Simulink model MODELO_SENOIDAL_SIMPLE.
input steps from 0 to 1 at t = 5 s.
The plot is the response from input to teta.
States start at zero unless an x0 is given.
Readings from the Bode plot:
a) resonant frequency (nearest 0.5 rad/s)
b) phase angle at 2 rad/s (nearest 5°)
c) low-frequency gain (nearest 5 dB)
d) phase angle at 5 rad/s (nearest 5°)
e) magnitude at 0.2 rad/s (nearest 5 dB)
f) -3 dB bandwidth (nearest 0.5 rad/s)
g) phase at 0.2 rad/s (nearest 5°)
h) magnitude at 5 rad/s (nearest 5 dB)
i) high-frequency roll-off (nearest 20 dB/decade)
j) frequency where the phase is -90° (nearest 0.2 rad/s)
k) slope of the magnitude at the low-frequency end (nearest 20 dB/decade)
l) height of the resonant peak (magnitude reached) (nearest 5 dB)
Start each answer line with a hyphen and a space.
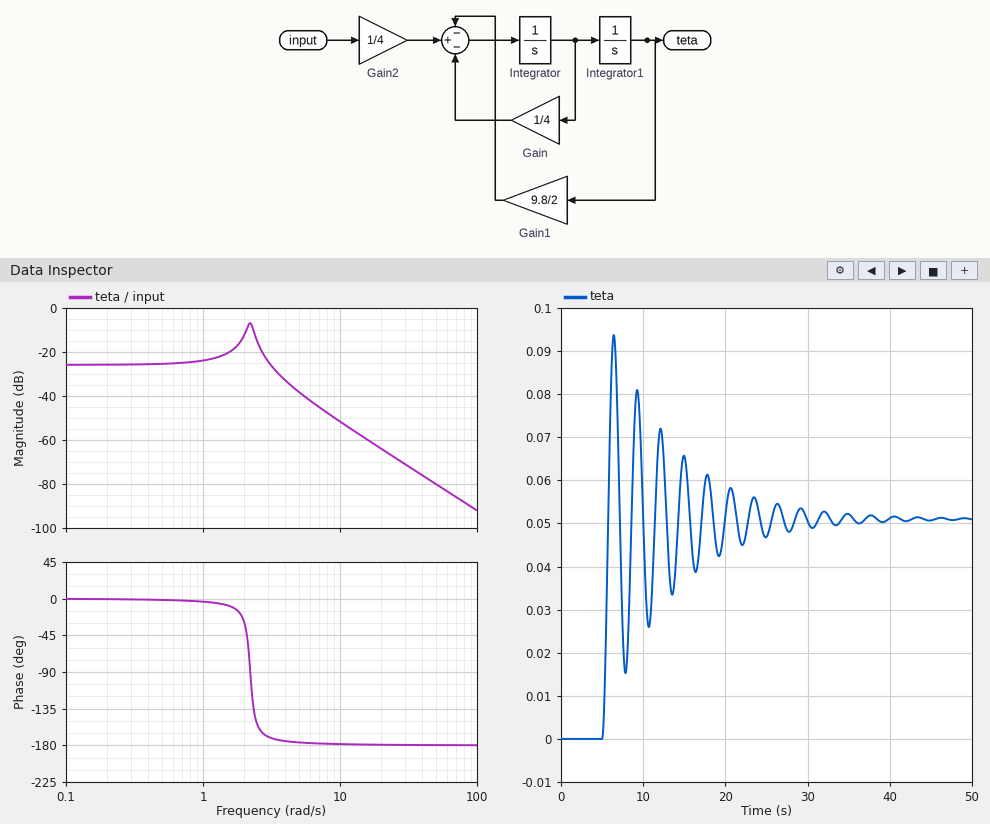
- 2.0 rad/s
- -30°
- -25 dB
- -175°
- -25 dB
- 3.5 rad/s
- 0°
- -40 dB
- -40 dB/decade
- 2.2 rad/s
- 0 dB/decade
- -5 dB
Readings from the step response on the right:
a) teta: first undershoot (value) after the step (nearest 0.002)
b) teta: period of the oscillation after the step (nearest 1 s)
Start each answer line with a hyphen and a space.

- 0.016
- 3 s
